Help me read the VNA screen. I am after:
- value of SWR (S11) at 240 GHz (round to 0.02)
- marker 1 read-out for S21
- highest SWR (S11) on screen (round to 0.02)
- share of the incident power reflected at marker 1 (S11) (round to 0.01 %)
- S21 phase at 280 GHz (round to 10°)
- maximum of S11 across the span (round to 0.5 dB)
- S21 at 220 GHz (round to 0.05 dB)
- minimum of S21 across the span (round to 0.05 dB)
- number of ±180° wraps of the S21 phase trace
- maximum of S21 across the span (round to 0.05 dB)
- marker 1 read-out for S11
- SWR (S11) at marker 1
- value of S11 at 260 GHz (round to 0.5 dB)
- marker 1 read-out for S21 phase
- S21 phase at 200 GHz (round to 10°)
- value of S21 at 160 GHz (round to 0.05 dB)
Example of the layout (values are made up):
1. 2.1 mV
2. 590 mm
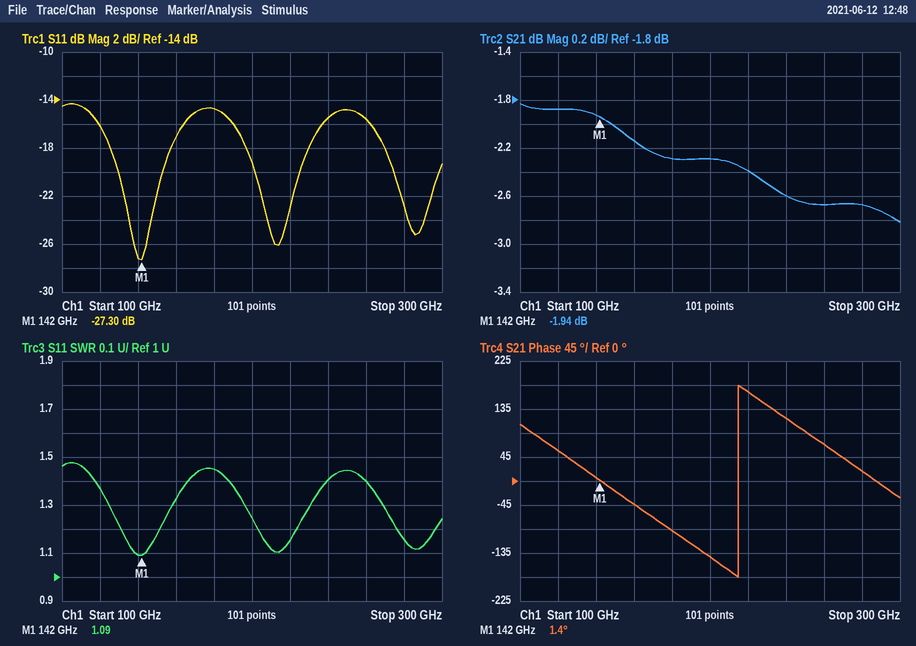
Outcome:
1. 1.40
2. -1.94 dB
3. 1.48
4. 0.19 %
5. 20°
6. -14.5 dB
7. -2.40 dB
8. -2.80 dB
9. 1
10. -1.85 dB
11. -27.30 dB
12. 1.09
13. -15.5 dB
14. 1.4°
15. -140°
16. -2.15 dB
